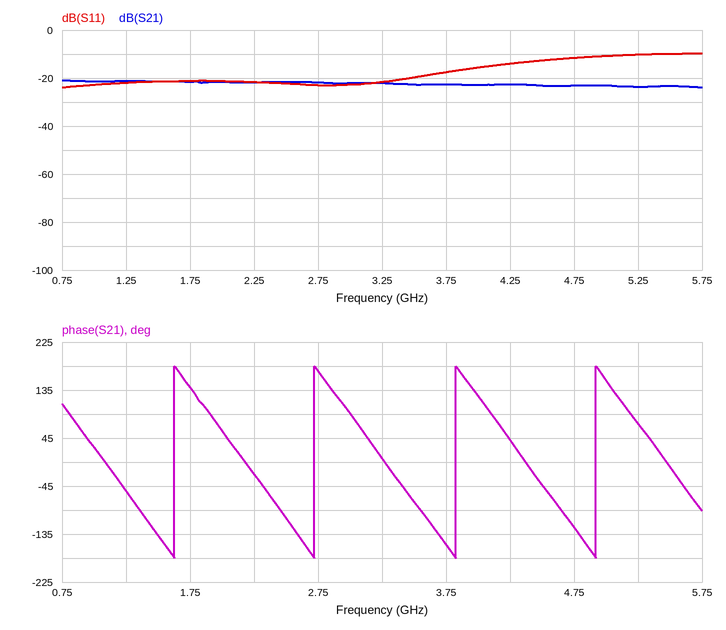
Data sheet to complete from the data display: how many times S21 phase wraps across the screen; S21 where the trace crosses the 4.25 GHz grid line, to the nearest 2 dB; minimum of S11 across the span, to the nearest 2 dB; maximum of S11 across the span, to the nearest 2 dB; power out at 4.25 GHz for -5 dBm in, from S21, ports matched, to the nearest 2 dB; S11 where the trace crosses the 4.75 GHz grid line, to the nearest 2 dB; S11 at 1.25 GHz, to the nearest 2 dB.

4
-22 dB
-24 dB
-10 dB
-28 dBm
-12 dB
-22 dB
